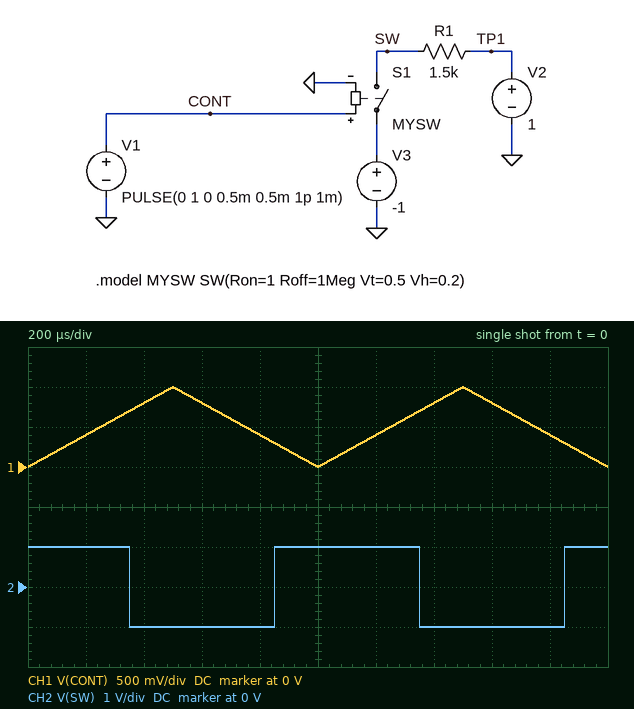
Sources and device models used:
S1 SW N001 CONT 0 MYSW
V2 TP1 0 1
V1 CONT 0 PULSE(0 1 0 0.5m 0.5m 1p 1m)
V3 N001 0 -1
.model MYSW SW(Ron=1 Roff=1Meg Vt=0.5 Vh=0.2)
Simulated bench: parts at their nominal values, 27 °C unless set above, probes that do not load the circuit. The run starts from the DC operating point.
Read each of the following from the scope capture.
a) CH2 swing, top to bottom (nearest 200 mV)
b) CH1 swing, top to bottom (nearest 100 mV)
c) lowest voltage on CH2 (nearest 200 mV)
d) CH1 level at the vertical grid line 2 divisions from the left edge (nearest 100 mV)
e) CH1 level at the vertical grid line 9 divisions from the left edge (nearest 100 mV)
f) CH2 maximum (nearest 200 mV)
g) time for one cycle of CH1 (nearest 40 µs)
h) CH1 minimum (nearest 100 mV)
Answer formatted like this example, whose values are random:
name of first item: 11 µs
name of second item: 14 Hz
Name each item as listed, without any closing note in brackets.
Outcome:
CH2 swing, top to bottom: 2.0 V
CH1 swing, top to bottom: 1.0 V
lowest voltage on CH2: -1.0 V
CH1 level at the vertical grid line 2 divisions from the left edge: 800 mV
CH1 level at the vertical grid line 9 divisions from the left edge: 400 mV
CH2 maximum: 1.0 V
time for one cycle of CH1: 1.00 ms
CH1 minimum: 0 V
